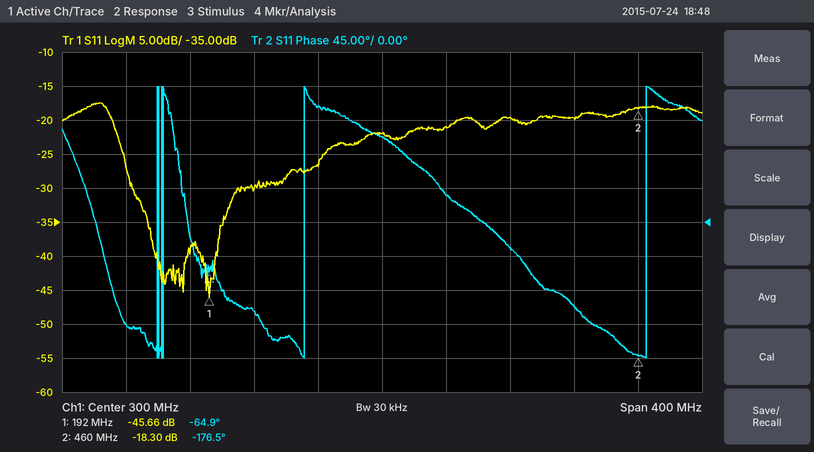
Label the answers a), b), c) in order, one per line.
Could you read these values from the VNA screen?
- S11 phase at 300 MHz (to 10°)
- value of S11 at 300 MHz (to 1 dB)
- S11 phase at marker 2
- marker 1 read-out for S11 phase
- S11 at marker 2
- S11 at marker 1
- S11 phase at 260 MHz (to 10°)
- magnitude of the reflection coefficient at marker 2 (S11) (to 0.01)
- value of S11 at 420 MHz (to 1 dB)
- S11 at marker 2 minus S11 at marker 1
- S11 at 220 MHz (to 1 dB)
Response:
a) 110°
b) -22 dB
c) -176.5°
d) -64.9°
e) -18.30 dB
f) -45.66 dB
g) 150°
h) 0.12
i) -20 dB
j) 27.36 dB
k) -30 dB
